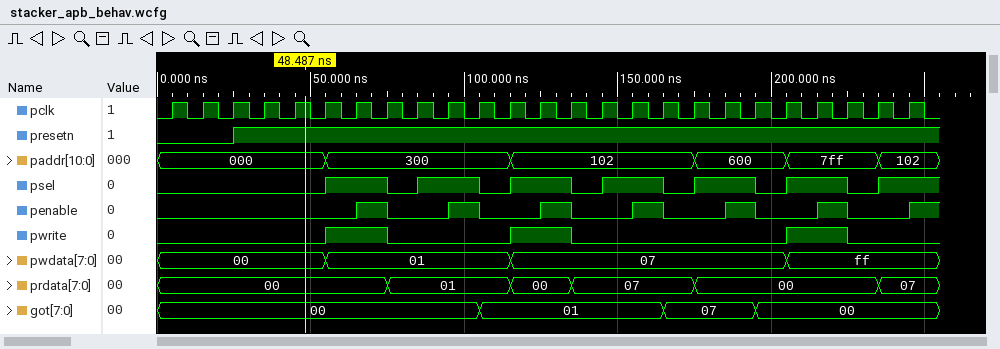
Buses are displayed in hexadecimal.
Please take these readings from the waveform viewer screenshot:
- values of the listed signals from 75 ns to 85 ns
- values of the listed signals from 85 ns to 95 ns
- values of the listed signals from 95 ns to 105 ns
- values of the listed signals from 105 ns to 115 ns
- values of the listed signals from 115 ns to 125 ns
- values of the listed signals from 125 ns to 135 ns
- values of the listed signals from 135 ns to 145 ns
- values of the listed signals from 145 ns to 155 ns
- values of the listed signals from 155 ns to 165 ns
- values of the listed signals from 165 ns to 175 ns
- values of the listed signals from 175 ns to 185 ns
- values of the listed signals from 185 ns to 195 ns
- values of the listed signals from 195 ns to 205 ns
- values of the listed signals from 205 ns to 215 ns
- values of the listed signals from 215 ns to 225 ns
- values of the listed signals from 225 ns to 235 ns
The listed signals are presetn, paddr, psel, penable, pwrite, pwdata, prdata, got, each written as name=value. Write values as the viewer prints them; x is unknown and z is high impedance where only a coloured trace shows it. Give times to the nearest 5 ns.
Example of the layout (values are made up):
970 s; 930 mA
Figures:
presetn=1, paddr=300, psel=0, penable=0, pwrite=0, pwdata=01, prdata=01, got=00; presetn=1, paddr=300, psel=1, penable=0, pwrite=0, pwdata=01, prdata=01, got=00; presetn=1, paddr=300, psel=1, penable=1, pwrite=0, pwdata=01, prdata=01, got=00; presetn=1, paddr=300, psel=0, penable=0, pwrite=0, pwdata=01, prdata=01, got=01; presetn=1, paddr=102, psel=1, penable=0, pwrite=1, pwdata=07, prdata=00, got=01; presetn=1, paddr=102, psel=1, penable=1, pwrite=1, pwdata=07, prdata=00, got=01; presetn=1, paddr=102, psel=0, penable=0, pwrite=0, pwdata=07, prdata=07, got=01; presetn=1, paddr=102, psel=1, penable=0, pwrite=0, pwdata=07, prdata=07, got=01; presetn=1, paddr=102, psel=1, penable=1, pwrite=0, pwdata=07, prdata=07, got=01; presetn=1, paddr=102, psel=0, penable=0, pwrite=0, pwdata=07, prdata=07, got=07; presetn=1, paddr=600, psel=1, penable=0, pwrite=0, pwdata=07, prdata=00, got=07; presetn=1, paddr=600, psel=1, penable=1, pwrite=0, pwdata=07, prdata=00, got=07; presetn=1, paddr=600, psel=0, penable=0, pwrite=0, pwdata=07, prdata=00, got=00; presetn=1, paddr=7ff, psel=1, penable=0, pwrite=1, pwdata=ff, prdata=00, got=00; presetn=1, paddr=7ff, psel=1, penable=1, pwrite=1, pwdata=ff, prdata=00, got=00; presetn=1, paddr=7ff, psel=0, penable=0, pwrite=0, pwdata=ff, prdata=00, got=00
